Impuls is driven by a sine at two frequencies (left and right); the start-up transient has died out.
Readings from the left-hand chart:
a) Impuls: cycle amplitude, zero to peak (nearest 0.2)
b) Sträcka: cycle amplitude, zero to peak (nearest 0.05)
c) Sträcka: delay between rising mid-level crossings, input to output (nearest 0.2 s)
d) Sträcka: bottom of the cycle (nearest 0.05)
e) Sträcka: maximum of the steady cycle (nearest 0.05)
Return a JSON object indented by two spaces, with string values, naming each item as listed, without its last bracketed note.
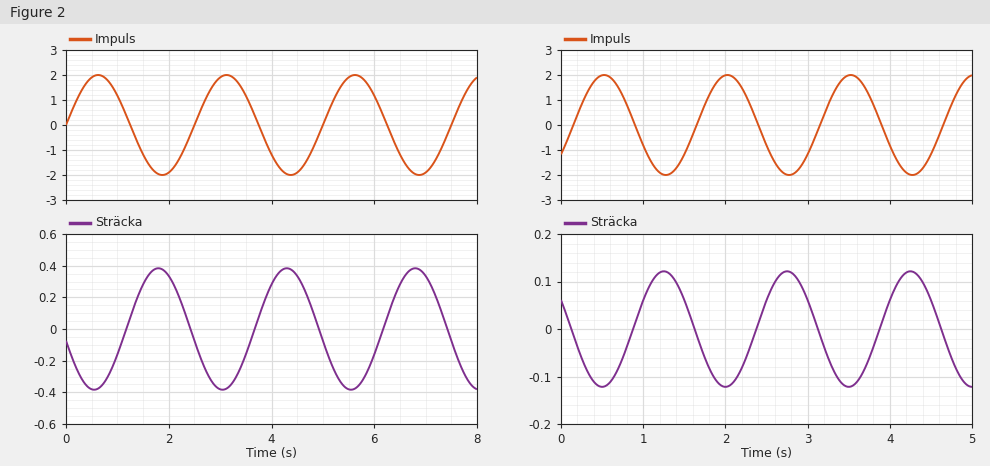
{
  "Impuls: cycle amplitude, zero to peak": "2.0",
  "Sträcka: cycle amplitude, zero to peak": "0.40",
  "Sträcka: delay between rising mid-level crossings, input to output": "1.2 s",
  "Sträcka: bottom of the cycle": "-0.40",
  "Sträcka: maximum of the steady cycle": "0.40"
}
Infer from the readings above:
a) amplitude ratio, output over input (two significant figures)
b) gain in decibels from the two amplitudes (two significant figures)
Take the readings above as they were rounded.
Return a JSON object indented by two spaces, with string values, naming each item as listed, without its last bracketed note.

{
  "amplitude ratio, output over input": "0.20",
  "gain in decibels from the two amplitudes": "-14 dB"
}
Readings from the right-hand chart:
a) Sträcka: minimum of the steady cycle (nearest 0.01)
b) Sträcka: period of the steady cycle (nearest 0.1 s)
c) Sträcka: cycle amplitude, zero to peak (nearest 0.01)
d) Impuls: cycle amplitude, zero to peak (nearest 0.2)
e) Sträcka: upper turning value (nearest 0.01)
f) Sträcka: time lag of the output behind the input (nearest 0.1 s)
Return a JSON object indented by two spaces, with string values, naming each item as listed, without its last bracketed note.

{
  "Sträcka: minimum of the steady cycle": "-0.12",
  "Sträcka: period of the steady cycle": "1.5 s",
  "Sträcka: cycle amplitude, zero to peak": "0.12",
  "Impuls: cycle amplitude, zero to peak": "2.0",
  "Sträcka: upper turning value": "0.12",
  "Sträcka: time lag of the output behind the input": "0.7 s"
}
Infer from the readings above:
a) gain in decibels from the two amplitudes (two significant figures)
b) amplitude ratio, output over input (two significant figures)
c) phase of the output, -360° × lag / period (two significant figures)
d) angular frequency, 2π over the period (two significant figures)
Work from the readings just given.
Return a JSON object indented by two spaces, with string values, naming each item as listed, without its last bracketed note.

{
  "gain in decibels from the two amplitudes": "-24 dB",
  "amplitude ratio, output over input": "0.060",
  "phase of the output, -360° × lag / period": "-170°",
  "angular frequency, 2π over the period": "4.2 rad/s"
}
